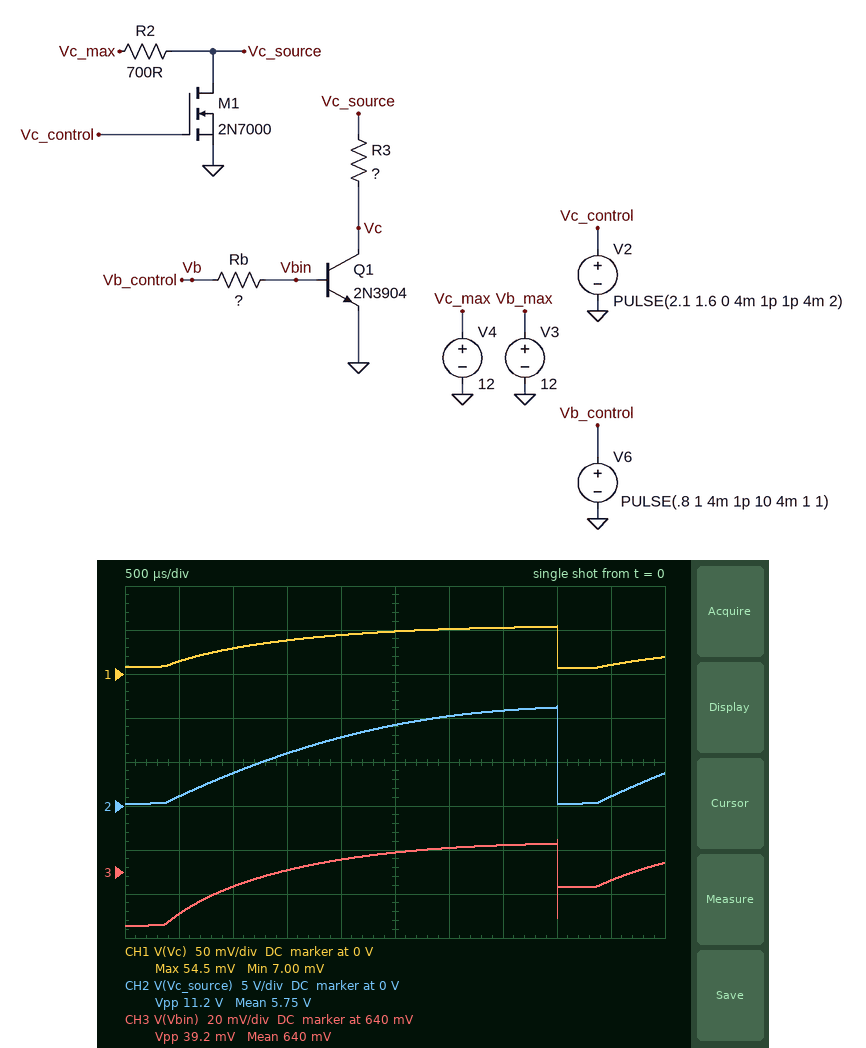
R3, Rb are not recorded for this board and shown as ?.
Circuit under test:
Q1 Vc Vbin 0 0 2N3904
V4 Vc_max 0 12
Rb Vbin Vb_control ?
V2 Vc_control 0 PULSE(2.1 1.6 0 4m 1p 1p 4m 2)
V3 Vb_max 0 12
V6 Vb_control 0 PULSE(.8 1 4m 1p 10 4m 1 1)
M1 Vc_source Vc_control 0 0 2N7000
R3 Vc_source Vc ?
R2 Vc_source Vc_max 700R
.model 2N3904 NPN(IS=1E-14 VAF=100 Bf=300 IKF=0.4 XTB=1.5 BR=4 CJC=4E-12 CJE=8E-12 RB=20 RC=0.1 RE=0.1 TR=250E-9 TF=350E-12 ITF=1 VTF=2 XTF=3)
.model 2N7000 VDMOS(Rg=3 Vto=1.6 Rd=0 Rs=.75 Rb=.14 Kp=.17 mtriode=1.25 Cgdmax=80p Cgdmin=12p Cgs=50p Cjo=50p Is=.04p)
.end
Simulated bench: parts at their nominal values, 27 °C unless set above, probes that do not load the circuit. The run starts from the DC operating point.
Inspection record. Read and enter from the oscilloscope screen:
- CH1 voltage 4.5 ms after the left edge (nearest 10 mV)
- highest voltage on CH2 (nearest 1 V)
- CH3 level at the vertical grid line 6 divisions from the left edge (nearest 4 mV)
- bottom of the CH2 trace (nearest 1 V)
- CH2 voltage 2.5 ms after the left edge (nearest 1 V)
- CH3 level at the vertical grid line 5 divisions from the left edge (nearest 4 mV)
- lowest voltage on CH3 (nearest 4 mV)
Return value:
10 mV
11 V
652 mV
0 V
9 V
648 mV
616 mV
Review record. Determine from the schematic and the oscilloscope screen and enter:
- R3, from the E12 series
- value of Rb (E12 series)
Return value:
15 kΩ
4.7 kΩ
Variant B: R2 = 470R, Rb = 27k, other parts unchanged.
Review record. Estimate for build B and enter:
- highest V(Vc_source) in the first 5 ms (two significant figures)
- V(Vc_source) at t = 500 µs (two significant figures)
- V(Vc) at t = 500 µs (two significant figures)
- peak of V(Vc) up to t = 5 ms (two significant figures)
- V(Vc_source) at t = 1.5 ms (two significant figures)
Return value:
12 V
4.6 V
71 mV
110 mV
7.9 V
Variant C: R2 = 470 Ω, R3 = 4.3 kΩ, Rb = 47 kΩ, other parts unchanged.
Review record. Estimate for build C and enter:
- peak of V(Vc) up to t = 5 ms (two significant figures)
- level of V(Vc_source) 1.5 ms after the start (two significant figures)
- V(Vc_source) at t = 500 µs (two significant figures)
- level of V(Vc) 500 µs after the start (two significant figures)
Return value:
7.1 V
7.7 V
4.3 V
270 mV
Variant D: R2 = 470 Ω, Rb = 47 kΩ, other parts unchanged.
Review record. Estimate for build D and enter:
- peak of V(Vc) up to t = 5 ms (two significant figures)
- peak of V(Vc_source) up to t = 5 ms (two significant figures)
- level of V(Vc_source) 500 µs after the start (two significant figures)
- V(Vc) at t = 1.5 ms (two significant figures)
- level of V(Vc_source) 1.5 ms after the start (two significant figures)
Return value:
150 mV
12 V
4.6 V
110 mV
7.9 V
